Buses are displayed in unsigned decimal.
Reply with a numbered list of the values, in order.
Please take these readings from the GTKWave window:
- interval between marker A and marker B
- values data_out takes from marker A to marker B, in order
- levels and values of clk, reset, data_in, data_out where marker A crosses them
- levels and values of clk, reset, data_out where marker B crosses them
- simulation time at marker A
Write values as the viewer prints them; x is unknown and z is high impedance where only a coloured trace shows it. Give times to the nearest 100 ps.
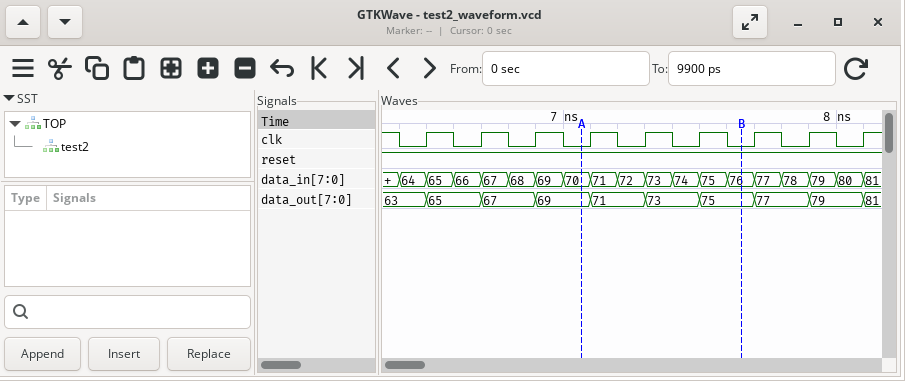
1. 600 ps
2. 69, 71, 73, 75
3. clk=0, reset=1, data_in=70, data_out=69
4. clk=0, reset=1, data_out=75
5. 7100 ps
